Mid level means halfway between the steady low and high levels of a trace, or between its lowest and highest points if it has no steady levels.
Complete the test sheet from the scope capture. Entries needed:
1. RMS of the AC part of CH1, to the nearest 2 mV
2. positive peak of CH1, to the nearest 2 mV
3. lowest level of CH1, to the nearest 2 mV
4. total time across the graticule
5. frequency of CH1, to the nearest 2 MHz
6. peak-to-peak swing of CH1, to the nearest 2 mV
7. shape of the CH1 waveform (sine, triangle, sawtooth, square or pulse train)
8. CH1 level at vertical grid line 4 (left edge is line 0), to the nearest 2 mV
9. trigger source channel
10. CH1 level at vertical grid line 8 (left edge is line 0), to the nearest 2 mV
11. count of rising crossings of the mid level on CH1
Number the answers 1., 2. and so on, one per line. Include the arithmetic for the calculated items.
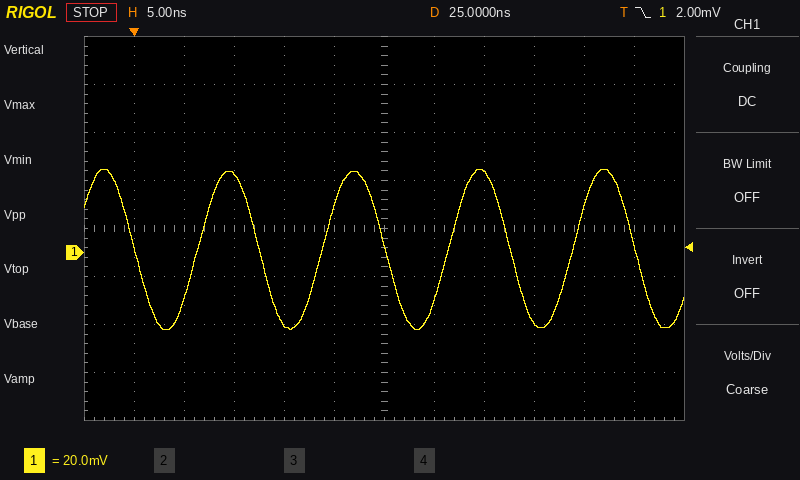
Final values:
1. 66 mV / (2√2) ≈ 23.3 mV, so 24 mV to the nearest 2 mV
2. 34 mV
3. -32 mV
4. 60 ns
5. 80 MHz
6. 34 mV − (-32 mV) = 66 mV
7. sine
8. -30 mV
9. CH1
10. 34 mV
11. 4
